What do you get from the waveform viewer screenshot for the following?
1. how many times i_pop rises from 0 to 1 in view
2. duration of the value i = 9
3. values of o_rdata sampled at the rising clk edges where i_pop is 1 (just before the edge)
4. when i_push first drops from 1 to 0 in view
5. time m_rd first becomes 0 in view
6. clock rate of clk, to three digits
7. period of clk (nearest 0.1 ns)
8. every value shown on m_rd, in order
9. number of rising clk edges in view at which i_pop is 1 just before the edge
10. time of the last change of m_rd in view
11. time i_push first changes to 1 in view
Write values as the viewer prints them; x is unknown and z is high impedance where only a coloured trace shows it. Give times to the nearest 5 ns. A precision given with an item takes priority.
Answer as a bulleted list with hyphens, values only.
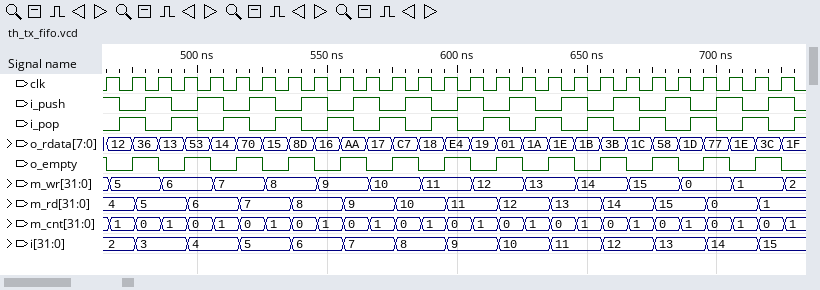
- 14
- 20 ns
- 12, 13, 14, 15, 16, 17, 18, 19, 1A, 1B, 1C, 1D, 1E
- 470 ns
- 695 ns
- 100 MHz
- 10 ns
- 4, 5, 6, 7, 8, 9, 10, 11, 12, 13, 14, 15, 0, 1
- 13
- 715 ns
- 480 ns
